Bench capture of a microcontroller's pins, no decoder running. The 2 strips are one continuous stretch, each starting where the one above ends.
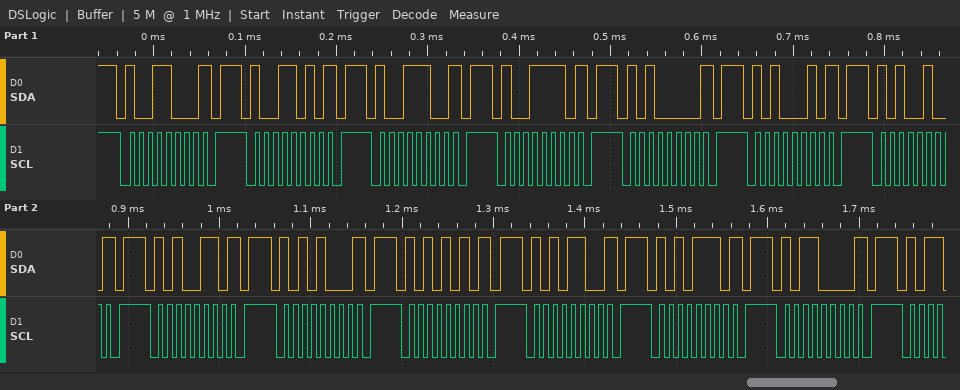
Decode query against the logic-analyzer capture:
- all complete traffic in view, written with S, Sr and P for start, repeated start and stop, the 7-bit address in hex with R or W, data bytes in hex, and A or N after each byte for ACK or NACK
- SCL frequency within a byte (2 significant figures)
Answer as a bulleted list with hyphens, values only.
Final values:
- S 4CW N P S 4DW N P S 4EW N P S 4FW N P S 50W N P S 51W N P S 52W N P S 53W N P S 54W N P S 55W N P S 56W N P S 57W N P S 58W N P
- 100 kHz
